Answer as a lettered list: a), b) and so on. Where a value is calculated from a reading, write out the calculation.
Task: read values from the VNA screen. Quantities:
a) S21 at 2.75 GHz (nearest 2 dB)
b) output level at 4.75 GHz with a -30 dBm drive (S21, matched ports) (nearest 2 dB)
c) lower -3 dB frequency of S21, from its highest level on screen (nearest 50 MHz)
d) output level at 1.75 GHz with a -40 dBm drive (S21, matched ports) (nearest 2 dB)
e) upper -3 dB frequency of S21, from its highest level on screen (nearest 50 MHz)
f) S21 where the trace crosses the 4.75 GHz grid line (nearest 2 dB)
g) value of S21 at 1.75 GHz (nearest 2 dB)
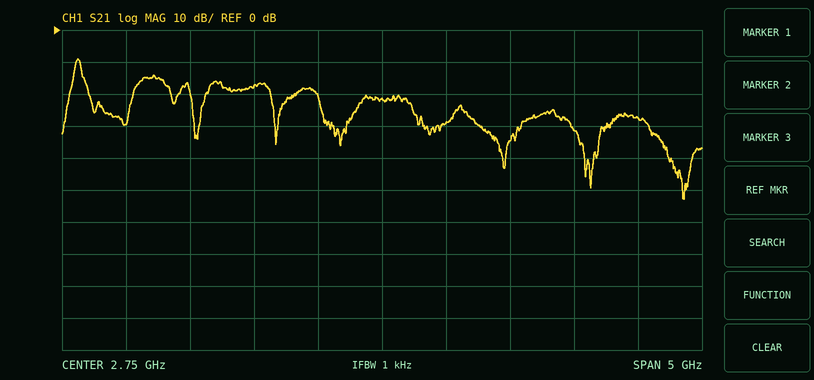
a) -22 dB
b) -30 dBm + (-28 dB) = -58 dBm
c) 350 MHz
d) -40 dBm + (-18 dB) = -58 dBm
e) 400 MHz
f) -28 dB
g) -18 dB
